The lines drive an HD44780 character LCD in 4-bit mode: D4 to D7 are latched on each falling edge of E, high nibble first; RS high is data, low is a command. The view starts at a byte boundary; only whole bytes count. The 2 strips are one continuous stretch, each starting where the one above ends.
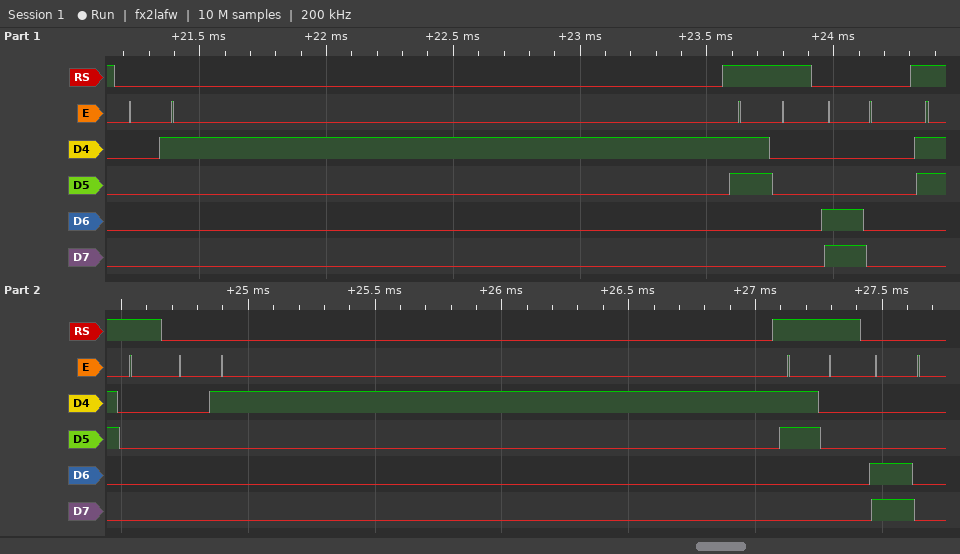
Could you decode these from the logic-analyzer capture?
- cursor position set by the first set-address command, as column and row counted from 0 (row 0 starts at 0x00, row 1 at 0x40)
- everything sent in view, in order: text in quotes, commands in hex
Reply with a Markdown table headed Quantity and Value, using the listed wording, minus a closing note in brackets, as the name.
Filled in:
| Quantity | Value |
|---|---|
| cursor position set by the first set-address command, as column and row counted from 0 | column 0, row 1 |
| everything sent in view, in order: text in quotes, commands in hex | 0x01 "0" 0xC0 "0" 0x01 "0" 0xC0 |
